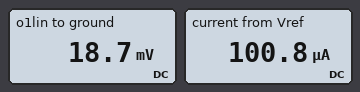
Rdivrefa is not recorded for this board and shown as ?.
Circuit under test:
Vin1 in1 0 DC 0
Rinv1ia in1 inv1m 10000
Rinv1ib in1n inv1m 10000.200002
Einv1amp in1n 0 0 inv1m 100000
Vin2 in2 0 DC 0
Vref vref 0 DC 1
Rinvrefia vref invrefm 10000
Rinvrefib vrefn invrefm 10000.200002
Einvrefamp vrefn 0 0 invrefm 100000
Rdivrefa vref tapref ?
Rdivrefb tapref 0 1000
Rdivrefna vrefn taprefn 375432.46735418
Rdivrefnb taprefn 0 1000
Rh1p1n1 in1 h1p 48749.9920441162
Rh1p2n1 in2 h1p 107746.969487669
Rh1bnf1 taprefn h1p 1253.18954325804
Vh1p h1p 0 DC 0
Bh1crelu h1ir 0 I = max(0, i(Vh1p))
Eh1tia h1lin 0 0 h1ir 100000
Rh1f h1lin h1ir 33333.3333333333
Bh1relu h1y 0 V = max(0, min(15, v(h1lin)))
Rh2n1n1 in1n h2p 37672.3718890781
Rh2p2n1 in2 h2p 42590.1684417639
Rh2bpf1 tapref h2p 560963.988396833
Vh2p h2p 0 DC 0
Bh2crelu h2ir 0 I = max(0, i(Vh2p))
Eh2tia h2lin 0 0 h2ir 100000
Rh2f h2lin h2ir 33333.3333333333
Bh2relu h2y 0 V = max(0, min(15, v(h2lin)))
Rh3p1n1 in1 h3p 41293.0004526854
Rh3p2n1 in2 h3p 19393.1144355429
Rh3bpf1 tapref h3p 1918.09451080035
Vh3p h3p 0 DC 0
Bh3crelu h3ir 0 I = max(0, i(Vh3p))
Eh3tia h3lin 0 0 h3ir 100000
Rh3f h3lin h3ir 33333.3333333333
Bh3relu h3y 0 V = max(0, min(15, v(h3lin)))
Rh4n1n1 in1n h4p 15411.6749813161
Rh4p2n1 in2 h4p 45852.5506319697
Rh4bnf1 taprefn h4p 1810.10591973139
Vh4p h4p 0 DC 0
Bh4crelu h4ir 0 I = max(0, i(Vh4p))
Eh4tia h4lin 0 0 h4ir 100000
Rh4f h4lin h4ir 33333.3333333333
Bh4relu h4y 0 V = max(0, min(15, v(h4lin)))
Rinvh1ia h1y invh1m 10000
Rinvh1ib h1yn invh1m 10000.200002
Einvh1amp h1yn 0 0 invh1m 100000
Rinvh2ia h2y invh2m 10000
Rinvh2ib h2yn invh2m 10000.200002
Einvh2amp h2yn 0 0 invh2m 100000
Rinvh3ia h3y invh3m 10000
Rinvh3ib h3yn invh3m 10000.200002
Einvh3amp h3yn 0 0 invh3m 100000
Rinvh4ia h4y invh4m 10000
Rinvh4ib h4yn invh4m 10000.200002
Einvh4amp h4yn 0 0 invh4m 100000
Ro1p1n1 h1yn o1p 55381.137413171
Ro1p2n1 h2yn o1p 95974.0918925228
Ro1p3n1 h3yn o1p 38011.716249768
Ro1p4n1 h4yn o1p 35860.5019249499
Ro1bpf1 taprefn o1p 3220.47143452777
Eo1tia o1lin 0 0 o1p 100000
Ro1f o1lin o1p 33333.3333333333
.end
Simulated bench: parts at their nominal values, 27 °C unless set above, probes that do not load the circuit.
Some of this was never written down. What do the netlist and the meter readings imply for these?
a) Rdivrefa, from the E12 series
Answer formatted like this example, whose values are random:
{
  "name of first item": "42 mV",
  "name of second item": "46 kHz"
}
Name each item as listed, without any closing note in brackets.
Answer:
{
  "Rdivrefa, from the E12 series": "1.2 MΩ"
}
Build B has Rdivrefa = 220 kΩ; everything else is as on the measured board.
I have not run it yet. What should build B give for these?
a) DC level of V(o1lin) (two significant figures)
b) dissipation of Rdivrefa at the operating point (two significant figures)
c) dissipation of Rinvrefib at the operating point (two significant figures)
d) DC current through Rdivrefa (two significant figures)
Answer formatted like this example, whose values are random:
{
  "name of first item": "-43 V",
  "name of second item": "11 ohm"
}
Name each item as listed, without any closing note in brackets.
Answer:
{
  "DC level of V(o1lin)": "56 mV",
  "dissipation of Rdivrefa at the operating point": "4.5 µW",
  "dissipation of Rinvrefib at the operating point": "100 µW",
  "DC current through Rdivrefa": "4.5 µA"
}
